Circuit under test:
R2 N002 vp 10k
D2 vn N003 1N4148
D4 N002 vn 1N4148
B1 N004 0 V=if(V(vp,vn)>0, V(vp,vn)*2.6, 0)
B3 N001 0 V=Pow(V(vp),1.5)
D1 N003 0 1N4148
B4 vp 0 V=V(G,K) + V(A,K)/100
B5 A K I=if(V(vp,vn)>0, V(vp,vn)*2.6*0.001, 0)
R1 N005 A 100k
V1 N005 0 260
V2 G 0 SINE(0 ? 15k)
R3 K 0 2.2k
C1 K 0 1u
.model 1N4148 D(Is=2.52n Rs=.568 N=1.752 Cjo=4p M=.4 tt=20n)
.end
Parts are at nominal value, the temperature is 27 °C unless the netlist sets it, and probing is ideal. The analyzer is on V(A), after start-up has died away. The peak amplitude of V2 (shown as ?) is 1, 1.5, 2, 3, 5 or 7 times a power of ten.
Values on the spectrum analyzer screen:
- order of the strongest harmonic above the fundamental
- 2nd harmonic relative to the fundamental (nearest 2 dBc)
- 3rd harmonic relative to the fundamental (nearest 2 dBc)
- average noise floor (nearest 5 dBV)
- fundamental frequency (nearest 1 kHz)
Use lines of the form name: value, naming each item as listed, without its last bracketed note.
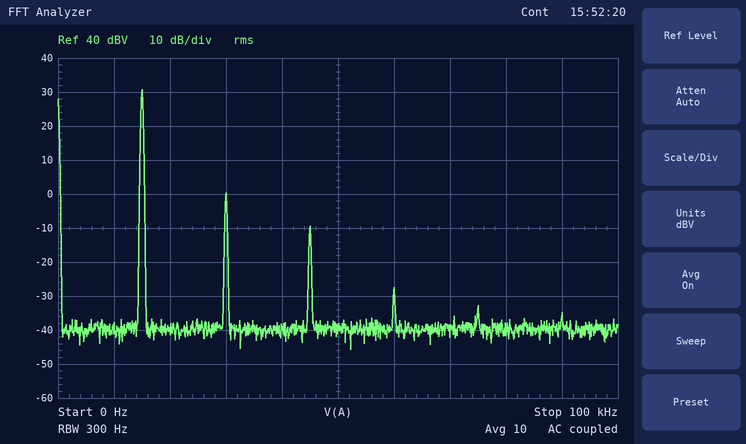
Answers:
order of the strongest harmonic above the fundamental: 2
2nd harmonic relative to the fundamental: -30 dBc
3rd harmonic relative to the fundamental: -40 dBc
average noise floor: -40 dBV
fundamental frequency: 15 kHz
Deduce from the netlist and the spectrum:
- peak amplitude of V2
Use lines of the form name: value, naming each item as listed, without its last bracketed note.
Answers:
peak amplitude of V2: 1 V
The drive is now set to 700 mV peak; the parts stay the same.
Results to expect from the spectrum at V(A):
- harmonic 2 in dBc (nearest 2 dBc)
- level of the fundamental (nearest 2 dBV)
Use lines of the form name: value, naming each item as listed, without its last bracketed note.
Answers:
harmonic 2 in dBc: -34 dBc
level of the fundamental: 28 dBV
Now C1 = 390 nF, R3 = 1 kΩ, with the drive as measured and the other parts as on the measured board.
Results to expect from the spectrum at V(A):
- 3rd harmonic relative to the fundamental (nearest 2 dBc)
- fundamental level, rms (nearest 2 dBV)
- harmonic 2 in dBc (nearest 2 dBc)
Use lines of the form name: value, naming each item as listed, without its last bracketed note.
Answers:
3rd harmonic relative to the fundamental: -44 dBc
fundamental level, rms: 32 dBV
harmonic 2 in dBc: -26 dBc
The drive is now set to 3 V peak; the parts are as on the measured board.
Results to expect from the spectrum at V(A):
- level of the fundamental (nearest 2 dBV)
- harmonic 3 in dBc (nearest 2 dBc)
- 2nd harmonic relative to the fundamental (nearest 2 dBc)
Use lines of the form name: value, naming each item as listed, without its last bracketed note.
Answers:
level of the fundamental: 38 dBV
harmonic 3 in dBc: -28 dBc
2nd harmonic relative to the fundamental: -10 dBc
